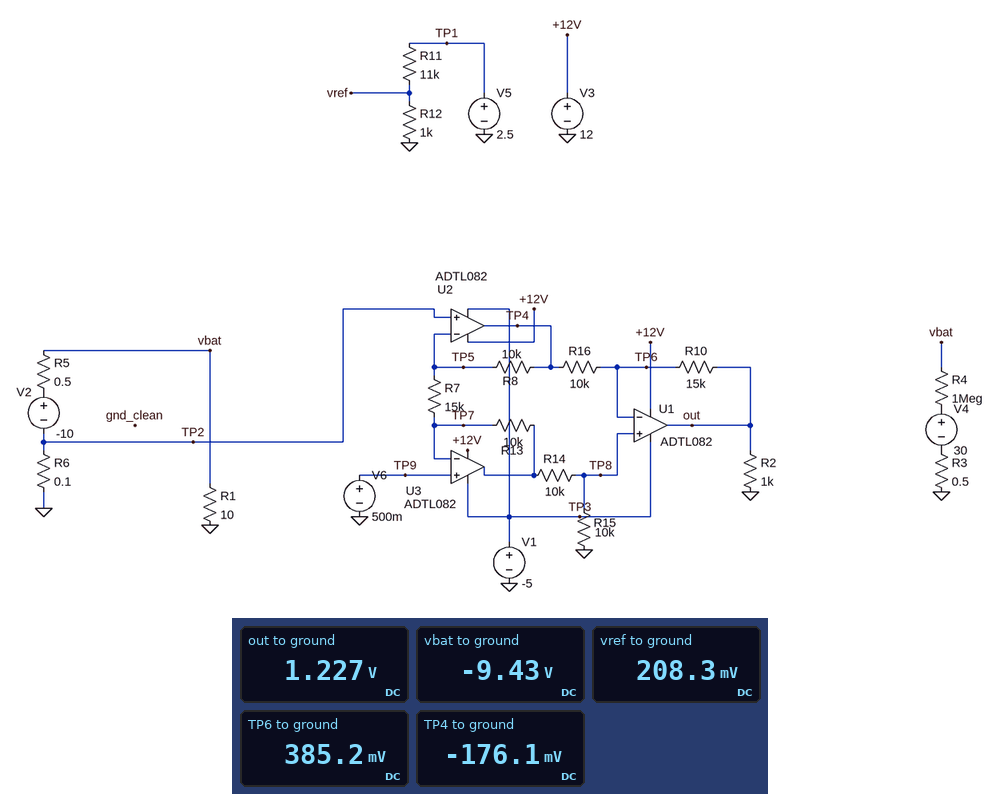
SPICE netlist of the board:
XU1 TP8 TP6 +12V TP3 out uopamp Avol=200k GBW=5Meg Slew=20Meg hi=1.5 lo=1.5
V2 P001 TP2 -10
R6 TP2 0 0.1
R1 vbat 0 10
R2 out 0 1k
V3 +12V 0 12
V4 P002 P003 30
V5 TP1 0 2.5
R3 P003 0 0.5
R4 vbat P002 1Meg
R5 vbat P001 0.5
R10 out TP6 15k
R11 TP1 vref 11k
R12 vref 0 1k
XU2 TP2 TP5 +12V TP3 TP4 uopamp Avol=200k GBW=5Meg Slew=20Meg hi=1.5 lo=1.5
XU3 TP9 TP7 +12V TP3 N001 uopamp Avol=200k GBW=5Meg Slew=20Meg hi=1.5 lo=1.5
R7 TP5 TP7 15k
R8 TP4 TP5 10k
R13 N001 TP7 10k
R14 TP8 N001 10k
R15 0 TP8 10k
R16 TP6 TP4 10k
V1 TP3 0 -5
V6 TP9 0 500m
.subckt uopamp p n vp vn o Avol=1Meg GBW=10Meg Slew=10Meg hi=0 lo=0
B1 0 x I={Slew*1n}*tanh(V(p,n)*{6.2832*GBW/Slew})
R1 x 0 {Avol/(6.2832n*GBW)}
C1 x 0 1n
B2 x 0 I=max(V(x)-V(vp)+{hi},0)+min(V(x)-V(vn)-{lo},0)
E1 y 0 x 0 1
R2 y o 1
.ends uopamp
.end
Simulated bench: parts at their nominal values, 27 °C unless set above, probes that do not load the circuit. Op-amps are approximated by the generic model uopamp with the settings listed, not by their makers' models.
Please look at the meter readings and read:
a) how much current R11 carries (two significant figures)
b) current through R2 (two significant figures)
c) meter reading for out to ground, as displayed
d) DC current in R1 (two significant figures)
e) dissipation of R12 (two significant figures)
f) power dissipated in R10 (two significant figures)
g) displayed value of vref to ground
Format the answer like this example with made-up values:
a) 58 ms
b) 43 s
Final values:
a) 210 µA
b) 1.2 mA
c) 1.227 V
d) 940 mA
e) 43 µW
f) 47 µW
g) 208.3 mV
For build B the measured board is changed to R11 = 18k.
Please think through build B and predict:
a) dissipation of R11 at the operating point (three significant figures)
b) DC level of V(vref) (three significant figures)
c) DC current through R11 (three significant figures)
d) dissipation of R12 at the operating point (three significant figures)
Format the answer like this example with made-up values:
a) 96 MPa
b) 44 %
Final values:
a) 312 µW
b) 132 mV
c) 132 µA
d) 17.3 µW
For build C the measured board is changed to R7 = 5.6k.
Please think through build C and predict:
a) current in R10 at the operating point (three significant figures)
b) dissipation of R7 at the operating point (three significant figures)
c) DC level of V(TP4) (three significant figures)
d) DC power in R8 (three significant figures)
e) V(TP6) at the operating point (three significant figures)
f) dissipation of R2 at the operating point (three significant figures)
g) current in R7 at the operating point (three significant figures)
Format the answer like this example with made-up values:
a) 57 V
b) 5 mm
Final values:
a) 124 µA
b) 29.4 µW
c) -630 mV
d) 52.5 µW
e) 612 mV
f) 6.13 mW
g) 72.4 µA
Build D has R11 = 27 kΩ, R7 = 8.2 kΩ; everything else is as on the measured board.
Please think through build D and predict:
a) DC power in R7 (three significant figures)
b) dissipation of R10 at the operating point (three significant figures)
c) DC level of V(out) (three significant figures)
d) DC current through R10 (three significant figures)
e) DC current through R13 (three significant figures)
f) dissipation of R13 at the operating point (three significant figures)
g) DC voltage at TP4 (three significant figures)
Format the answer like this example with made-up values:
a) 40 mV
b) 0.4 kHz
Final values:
a) 20.1 µW
b) 121 µW
c) 1.84 V
d) 89.8 µA
e) 49.5 µA
f) 24.5 µW
g) -400 mV
